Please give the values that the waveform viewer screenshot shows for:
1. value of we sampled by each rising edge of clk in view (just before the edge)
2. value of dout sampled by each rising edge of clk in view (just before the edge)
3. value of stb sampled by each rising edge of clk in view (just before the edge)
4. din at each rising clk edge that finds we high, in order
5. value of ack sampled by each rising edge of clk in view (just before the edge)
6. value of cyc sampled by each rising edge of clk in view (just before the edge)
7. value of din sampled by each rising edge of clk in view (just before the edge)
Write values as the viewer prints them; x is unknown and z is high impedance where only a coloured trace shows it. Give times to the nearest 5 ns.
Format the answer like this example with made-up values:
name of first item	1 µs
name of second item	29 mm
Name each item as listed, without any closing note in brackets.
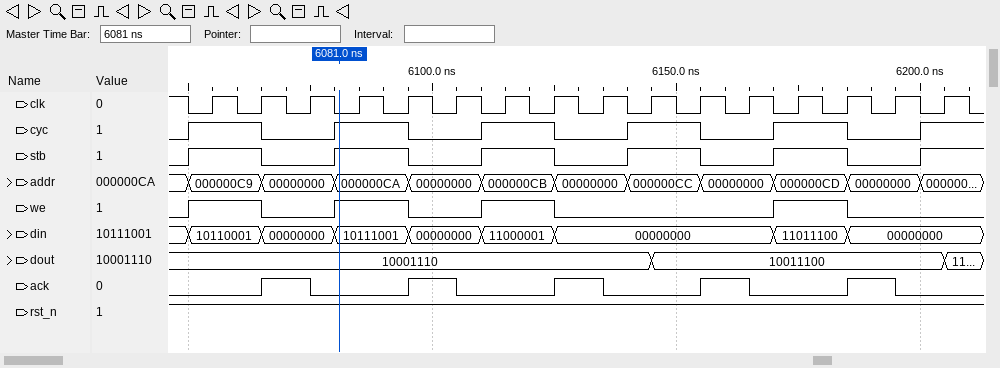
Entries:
value of we sampled by each rising edge of clk in view	1 1 0 1 1 0 1 1 0 0 0 0 1 1 0 0
value of dout sampled by each rising edge of clk in view	10001110, 10001110, 10001110, 10001110, 10001110, 10001110, 10001110, 10001110, 10001110, 10001110, 10011100, 10011100, 10011100, 10011100, 10011100, 10011100
value of stb sampled by each rising edge of clk in view	1 1 0 1 1 0 1 1 0 1 1 0 1 1 0 1
din at each rising clk edge that finds we high, in order	10110001, 10110001, 10111001, 10111001, 11000001, 11000001, 11011100, 11011100
value of ack sampled by each rising edge of clk in view	0 0 1 0 0 1 0 0 1 0 0 1 0 0 1 0
value of cyc sampled by each rising edge of clk in view	1 1 0 1 1 0 1 1 0 1 1 0 1 1 0 1
value of din sampled by each rising edge of clk in view	10110001, 10110001, 00000000, 10111001, 10111001, 00000000, 11000001, 11000001, 00000000, 00000000, 00000000, 00000000, 11011100, 11011100, 00000000, 00000000
